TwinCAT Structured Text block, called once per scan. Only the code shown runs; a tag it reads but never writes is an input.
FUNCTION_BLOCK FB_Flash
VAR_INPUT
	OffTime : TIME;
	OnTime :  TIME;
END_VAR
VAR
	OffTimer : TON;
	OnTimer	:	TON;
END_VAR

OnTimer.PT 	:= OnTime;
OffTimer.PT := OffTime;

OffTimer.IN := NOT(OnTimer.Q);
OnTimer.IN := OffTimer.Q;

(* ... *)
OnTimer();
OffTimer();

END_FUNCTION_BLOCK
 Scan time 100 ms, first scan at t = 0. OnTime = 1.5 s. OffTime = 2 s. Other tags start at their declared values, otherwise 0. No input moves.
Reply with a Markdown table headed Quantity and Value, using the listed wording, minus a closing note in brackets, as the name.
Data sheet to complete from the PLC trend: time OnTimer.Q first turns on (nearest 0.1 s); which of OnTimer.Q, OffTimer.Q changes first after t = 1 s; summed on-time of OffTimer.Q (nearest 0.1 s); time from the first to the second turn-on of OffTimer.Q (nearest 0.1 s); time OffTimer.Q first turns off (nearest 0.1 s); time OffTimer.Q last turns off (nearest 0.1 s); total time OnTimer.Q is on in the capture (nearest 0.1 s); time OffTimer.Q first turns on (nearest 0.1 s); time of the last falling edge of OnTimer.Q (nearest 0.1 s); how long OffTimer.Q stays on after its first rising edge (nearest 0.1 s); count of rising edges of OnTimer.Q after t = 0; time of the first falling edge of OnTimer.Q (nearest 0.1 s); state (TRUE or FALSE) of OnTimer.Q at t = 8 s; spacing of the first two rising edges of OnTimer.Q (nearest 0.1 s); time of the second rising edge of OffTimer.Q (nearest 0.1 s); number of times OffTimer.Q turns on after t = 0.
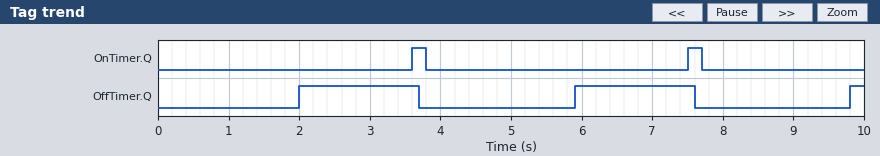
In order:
| Quantity | Value |
|---|---|
| time OnTimer.Q first turns on | 3.6 s |
| which of OnTimer.Q, OffTimer.Q changes first after t = 1 s | OffTimer.Q |
| summed on-time of OffTimer.Q | 3.6 s |
| time from the first to the second turn-on of OffTimer.Q | 3.9 s |
| time OffTimer.Q first turns off | 3.7 s |
| time OffTimer.Q last turns off | 7.6 s |
| total time OnTimer.Q is on in the capture | 0.4 s |
| time OffTimer.Q first turns on | 2.0 s |
| time of the last falling edge of OnTimer.Q | 7.7 s |
| how long OffTimer.Q stays on after its first rising edge | 1.7 s |
| count of rising edges of OnTimer.Q after t = 0 | 2 |
| time of the first falling edge of OnTimer.Q | 3.8 s |
| state (TRUE or FALSE) of OnTimer.Q at t = 8 s | FALSE |
| spacing of the first two rising edges of OnTimer.Q | 3.9 s |
| time of the second rising edge of OffTimer.Q | 5.9 s |
| number of times OffTimer.Q turns on after t = 0 | 3 |
